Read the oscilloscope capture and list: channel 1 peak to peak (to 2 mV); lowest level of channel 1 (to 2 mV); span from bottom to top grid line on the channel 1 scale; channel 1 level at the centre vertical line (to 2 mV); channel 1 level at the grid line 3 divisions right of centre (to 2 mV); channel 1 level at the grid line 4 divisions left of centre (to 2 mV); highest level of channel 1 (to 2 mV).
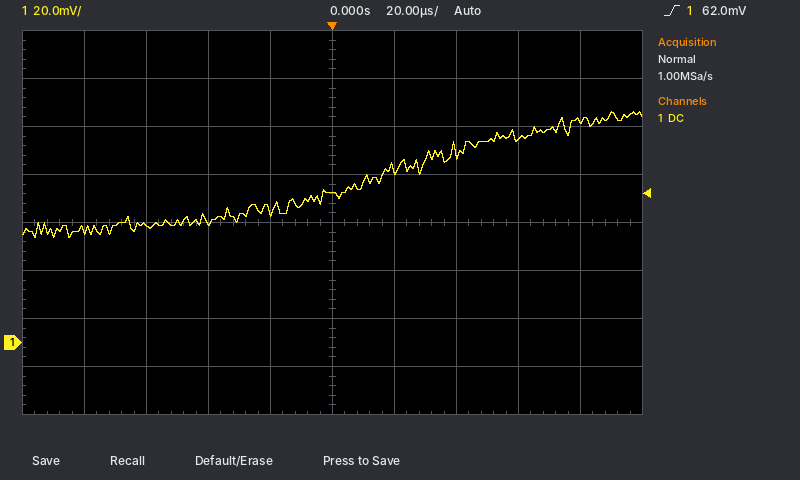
52 mV
44 mV
160 mV
62 mV
84 mV
46 mV
96 mV
